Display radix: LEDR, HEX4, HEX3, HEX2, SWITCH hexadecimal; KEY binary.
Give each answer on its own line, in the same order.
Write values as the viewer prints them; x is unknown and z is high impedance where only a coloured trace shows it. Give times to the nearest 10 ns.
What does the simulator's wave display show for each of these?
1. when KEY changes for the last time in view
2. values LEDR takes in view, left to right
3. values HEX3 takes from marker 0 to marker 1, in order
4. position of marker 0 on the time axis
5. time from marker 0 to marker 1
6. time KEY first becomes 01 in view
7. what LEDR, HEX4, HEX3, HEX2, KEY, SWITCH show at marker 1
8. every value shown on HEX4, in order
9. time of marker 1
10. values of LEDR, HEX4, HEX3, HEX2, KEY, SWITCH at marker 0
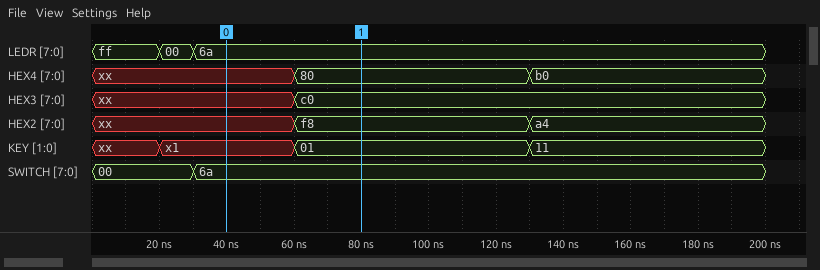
130 ns
ff, 00, 6a
xx, c0
40 ns
40 ns
60 ns
LEDR=6a, HEX4=80, HEX3=c0, HEX2=f8, KEY=01, SWITCH=6a
xx, 80, b0
80 ns
LEDR=6a, HEX4=xx, HEX3=xx, HEX2=xx, KEY=x1, SWITCH=6a
